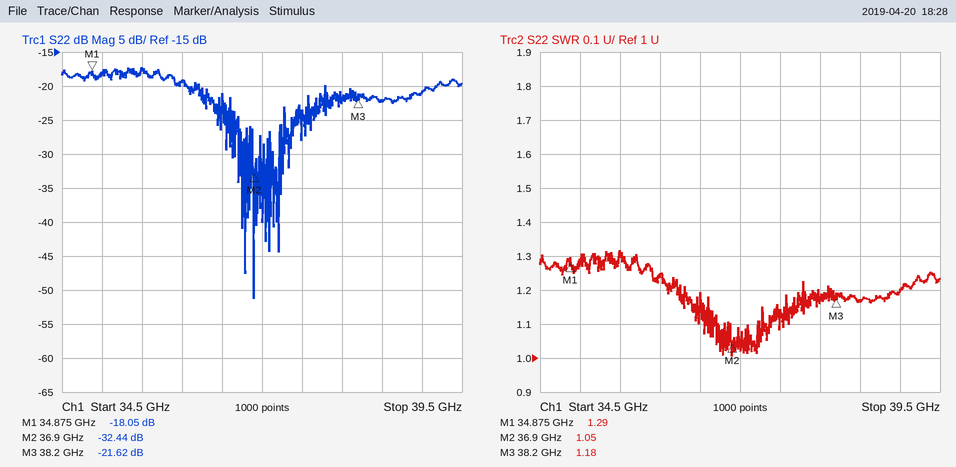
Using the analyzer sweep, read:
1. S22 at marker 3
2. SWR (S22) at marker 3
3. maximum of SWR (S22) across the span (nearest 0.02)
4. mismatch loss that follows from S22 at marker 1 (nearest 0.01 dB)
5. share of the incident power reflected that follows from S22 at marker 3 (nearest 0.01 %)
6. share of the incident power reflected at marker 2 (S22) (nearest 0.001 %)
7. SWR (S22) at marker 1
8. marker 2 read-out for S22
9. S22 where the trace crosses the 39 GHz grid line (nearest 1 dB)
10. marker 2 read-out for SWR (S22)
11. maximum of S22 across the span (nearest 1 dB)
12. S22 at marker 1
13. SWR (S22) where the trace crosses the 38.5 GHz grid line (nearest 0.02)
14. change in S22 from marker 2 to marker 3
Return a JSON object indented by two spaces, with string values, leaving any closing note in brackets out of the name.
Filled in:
{
  "S22 at marker 3": "-21.62 dB",
  "SWR (S22) at marker 3": "1.18",
  "maximum of SWR (S22) across the span": "1.32",
  "mismatch loss that follows from S22 at marker 1": "0.07 dB",
  "share of the incident power reflected that follows from S22 at marker 3": "0.69 %",
  "share of the incident power reflected at marker 2 (S22)": "0.057 %",
  "SWR (S22) at marker 1": "1.29",
  "marker 2 read-out for S22": "-32.44 dB",
  "S22 where the trace crosses the 39 GHz grid line": "-21 dB",
  "marker 2 read-out for SWR": "1.05",
  "maximum of S22 across the span": "-17 dB",
  "S22 at marker 1": "-18.05 dB",
  "SWR (S22) where the trace crosses the 38.5 GHz grid line": "1.16",
  "change in S22 from marker 2 to marker 3": "10.82 dB"
}
